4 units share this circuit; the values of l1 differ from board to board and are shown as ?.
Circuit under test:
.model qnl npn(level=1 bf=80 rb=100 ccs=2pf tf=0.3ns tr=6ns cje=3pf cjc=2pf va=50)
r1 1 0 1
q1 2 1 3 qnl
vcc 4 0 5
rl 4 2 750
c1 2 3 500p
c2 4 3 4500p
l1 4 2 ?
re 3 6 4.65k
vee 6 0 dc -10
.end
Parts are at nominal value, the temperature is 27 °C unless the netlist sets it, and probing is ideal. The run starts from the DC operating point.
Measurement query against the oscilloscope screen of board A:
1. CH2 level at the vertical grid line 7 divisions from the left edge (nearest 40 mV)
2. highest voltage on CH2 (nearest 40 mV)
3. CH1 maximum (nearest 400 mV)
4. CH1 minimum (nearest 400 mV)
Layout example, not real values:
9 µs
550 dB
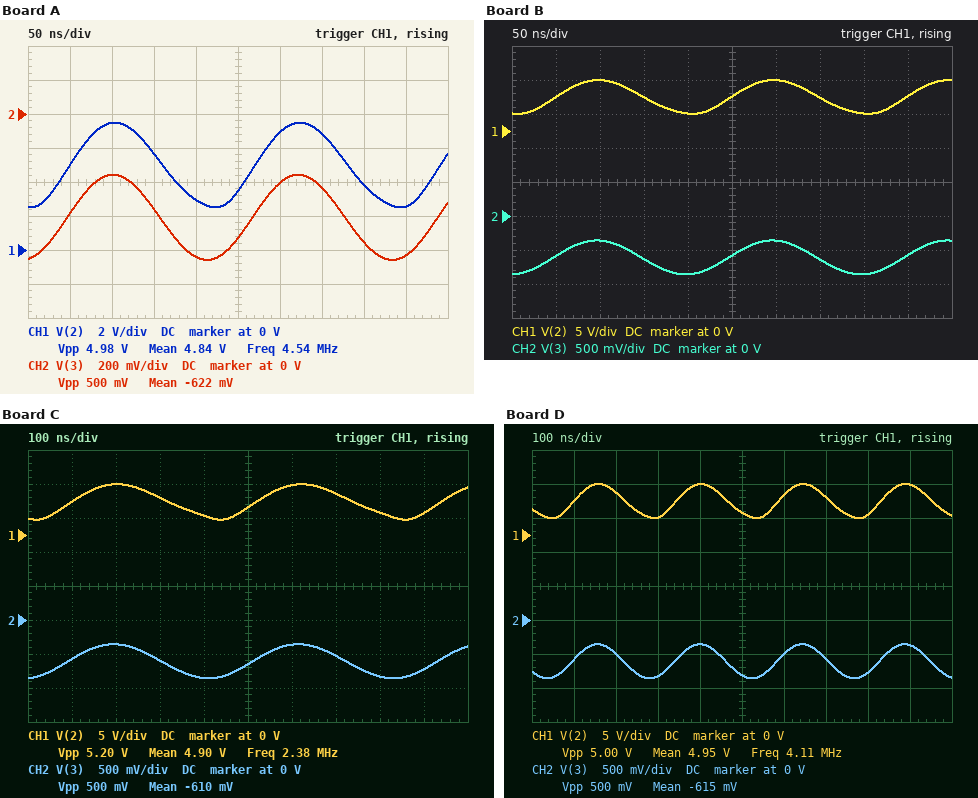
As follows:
-440 mV
-360 mV
7.6 V
2.4 V
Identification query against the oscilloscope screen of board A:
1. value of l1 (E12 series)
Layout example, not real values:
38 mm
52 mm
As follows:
2.7 µH
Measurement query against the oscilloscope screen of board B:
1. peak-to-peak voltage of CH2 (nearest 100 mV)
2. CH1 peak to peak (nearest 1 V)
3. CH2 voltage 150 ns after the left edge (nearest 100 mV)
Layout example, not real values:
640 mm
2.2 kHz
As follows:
500 mV
5 V
-600 mV
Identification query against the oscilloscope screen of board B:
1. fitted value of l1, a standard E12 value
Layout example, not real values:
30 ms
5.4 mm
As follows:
2.2 µH
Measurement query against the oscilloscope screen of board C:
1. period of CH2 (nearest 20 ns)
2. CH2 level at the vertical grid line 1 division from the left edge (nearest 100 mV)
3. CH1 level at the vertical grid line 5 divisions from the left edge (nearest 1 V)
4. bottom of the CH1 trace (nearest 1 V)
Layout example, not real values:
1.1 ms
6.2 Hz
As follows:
420 ns
-600 mV
4 V
2 V
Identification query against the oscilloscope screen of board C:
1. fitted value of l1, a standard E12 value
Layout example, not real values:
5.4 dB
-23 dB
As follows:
10 µH
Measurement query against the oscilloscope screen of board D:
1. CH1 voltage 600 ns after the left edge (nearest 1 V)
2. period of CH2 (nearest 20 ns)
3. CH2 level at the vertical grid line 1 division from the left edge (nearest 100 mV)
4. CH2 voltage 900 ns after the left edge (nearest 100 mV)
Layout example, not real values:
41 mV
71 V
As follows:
6 V
240 ns
-600 mV
-400 mV
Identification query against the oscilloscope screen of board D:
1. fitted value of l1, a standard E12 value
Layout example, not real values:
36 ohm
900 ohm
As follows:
3.3 µH
